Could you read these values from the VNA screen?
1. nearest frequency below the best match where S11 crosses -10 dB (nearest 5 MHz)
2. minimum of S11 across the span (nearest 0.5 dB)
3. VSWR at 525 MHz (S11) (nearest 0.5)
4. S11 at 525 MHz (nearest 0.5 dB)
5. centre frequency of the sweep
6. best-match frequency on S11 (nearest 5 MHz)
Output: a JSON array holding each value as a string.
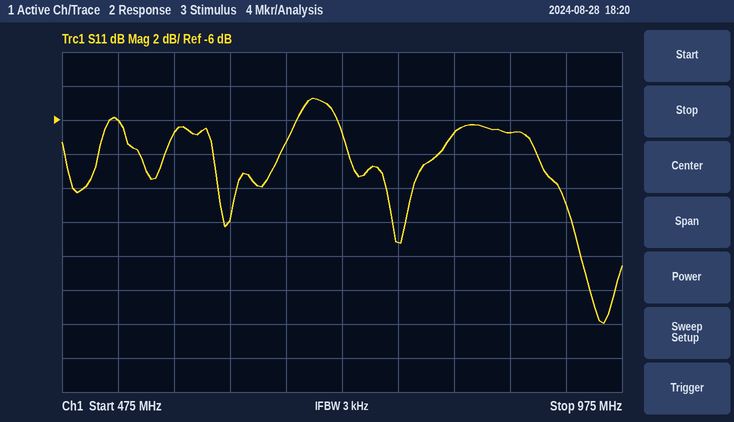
["920 MHz", "-18.0 dB", "3.0", "-6.0 dB", "725 MHz", "960 MHz"]
